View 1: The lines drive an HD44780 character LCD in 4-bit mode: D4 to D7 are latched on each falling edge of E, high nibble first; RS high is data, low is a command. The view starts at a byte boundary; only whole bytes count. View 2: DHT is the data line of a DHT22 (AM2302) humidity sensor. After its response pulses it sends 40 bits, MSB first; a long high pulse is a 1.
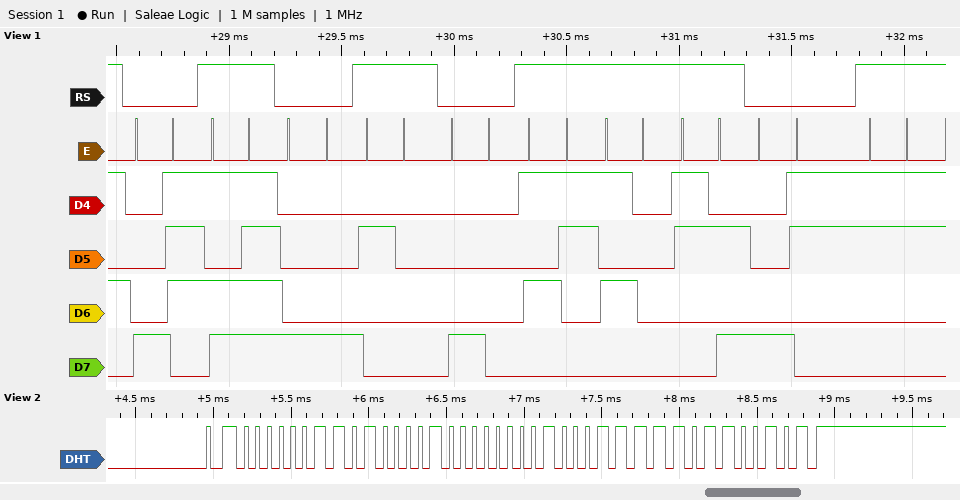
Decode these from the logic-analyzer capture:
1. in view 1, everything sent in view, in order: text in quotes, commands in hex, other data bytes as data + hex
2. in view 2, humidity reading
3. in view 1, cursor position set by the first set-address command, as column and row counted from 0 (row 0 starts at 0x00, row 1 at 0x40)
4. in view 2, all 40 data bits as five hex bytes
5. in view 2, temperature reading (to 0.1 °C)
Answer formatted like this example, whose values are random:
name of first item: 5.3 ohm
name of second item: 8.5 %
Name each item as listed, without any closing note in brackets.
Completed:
in view 1, everything sent in view, in order: text in quotes, commands in hex, other data bytes as data + hex: 0x87 data DF 0x88 " " 0x80 "SP:" 0x83 "3"
in view 2, humidity reading: 83.4 %
in view 1, cursor position set by the first set-address command, as column and row counted from 0: column 7, row 0
in view 2, all 40 data bits as five hex bytes: 03 42 01 1F 65
in view 2, temperature reading: 28.7 °C
